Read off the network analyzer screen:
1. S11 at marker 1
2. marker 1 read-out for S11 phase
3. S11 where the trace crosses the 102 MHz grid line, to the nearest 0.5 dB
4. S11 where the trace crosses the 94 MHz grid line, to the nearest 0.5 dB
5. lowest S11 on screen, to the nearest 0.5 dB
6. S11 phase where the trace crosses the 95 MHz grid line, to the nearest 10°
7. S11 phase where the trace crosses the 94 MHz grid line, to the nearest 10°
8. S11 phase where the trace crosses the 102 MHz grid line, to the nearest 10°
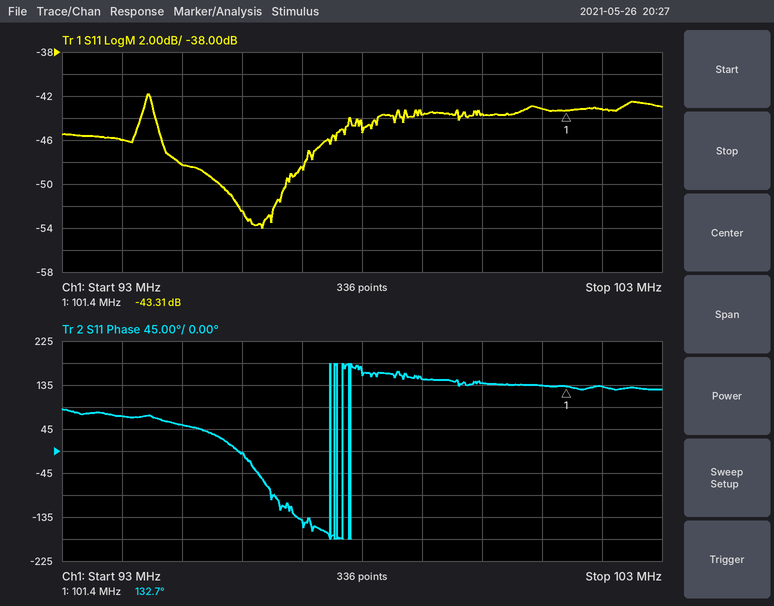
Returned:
-43.31 dB
132.7°
-43.0 dB
-46.0 dB
-54.0 dB
50°
70°
130°
